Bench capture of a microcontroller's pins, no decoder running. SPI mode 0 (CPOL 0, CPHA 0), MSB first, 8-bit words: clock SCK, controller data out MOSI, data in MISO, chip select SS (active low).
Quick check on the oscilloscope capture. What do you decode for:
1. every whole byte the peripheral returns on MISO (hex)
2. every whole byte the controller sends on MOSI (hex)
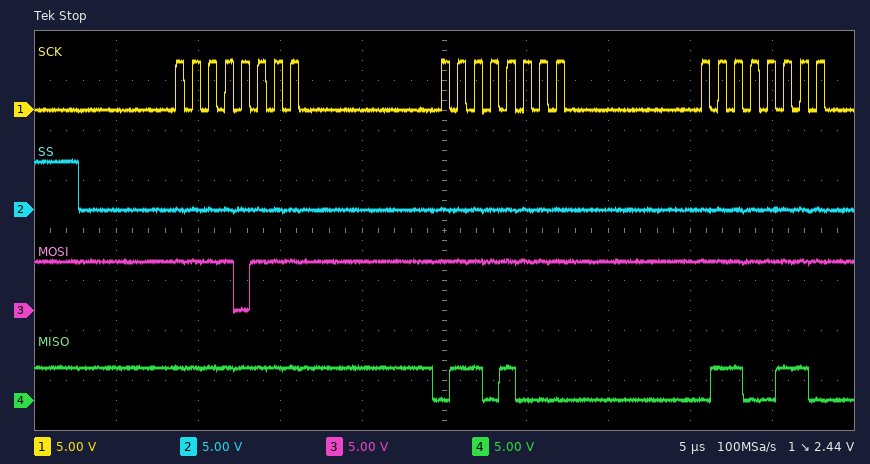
FF 68 66
F7 FF FF
